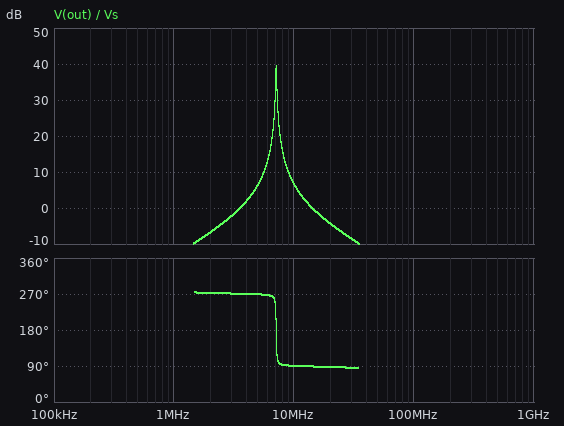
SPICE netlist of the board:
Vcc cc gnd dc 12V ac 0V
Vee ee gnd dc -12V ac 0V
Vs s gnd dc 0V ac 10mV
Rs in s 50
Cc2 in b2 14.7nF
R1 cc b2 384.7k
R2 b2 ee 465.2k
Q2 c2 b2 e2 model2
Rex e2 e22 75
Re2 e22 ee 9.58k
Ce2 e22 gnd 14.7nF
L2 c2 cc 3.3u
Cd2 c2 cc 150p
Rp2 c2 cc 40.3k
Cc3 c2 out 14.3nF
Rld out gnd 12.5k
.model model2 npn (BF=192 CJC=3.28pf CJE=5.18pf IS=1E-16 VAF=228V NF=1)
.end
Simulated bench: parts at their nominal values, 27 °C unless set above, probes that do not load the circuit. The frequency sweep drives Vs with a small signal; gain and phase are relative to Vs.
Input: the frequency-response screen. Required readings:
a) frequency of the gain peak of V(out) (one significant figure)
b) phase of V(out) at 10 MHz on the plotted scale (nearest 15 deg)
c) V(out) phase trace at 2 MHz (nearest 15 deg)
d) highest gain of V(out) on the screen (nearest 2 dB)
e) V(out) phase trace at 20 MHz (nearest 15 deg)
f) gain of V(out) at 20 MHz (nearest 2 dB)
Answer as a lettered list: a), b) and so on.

a) 7 MHz
b) 90 deg
c) 270 deg
d) 40 dB
e) 90 deg
f) -4 dB
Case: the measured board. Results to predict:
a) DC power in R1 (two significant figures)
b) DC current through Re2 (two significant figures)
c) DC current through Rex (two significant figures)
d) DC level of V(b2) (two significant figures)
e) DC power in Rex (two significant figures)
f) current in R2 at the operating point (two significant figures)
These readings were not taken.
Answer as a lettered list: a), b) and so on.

a) 380 µW
b) 1.2 mA
c) 1.2 mA
d) -62 mV
e) 100 µW
f) 26 µA
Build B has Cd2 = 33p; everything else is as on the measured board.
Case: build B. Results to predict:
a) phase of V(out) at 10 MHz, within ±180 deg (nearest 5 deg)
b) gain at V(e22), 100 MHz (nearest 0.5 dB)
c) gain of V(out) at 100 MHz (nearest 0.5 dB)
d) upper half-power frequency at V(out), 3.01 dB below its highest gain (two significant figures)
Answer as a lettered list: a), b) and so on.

a) -95 deg
b) -59.5 dB
c) -6.5 dB
d) 15 MHz
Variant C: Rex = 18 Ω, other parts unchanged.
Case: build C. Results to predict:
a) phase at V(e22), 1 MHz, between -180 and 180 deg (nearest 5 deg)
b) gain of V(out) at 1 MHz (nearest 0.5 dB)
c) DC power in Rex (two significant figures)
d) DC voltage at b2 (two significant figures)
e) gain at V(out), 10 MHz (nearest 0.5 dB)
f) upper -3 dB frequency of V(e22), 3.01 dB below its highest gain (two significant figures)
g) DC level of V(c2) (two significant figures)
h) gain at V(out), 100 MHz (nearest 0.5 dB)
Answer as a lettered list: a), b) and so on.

a) -75 deg
b) -6.0 dB
c) 24 µW
d) -68 mV
e) 14.0 dB
f) 270 kHz
g) 12 V
h) -12.0 dB
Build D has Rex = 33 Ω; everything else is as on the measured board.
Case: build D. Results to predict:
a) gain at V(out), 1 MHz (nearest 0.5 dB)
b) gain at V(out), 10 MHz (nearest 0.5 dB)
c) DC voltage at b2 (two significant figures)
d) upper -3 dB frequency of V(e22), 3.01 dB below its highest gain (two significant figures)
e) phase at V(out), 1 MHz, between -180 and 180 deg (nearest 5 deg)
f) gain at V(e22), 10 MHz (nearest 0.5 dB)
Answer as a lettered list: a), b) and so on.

a) -8.5 dB
b) 11.5 dB
c) -66 mV
d) 200 kHz
e) -80 deg
f) -34.5 dB
